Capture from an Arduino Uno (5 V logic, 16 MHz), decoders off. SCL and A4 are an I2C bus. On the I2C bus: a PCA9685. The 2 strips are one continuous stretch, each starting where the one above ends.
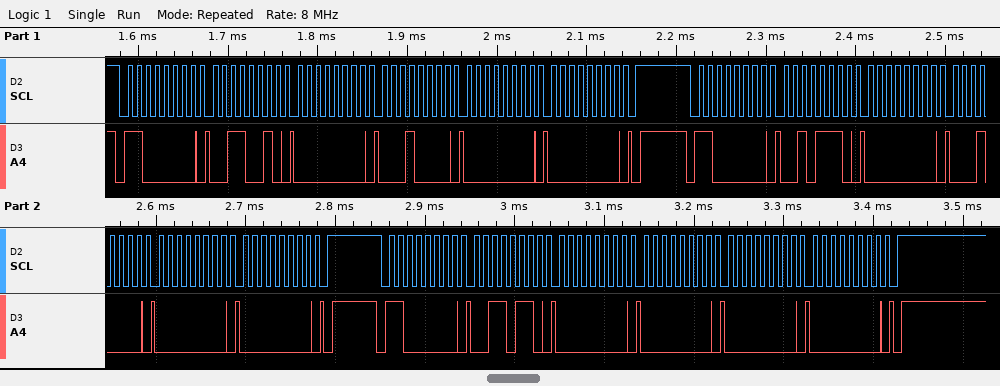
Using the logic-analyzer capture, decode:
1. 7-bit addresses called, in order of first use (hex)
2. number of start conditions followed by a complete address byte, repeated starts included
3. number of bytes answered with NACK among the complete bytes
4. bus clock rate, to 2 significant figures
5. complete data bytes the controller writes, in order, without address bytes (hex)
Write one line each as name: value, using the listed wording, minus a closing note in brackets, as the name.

7-bit addresses called, in order of first use: 0x60
number of start conditions followed by a complete address byte, repeated starts included: 3
number of bytes answered with NACK among the complete bytes: 0
bus clock rate, to 2 significant figures: 100 kHz
complete data bytes the controller writes, in order, without address bytes: 32 00 10 00 00 2E 00 10 00 00 36 00 00 00 00
